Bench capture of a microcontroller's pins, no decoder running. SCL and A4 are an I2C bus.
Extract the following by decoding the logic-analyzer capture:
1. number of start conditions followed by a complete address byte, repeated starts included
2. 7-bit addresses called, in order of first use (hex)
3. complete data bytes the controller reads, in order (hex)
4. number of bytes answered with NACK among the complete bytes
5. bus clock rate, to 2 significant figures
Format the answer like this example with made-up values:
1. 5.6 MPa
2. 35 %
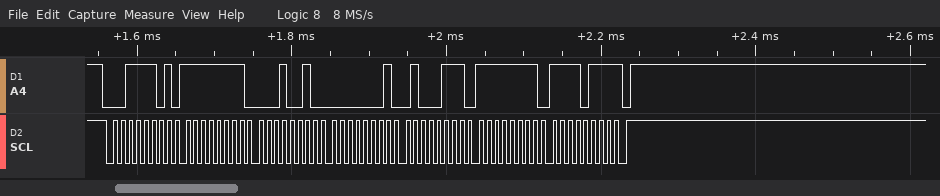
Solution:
1. 1
2. 0x1E
3. FF 12 01 47 FF F7
4. 1
5. 100 kHz
